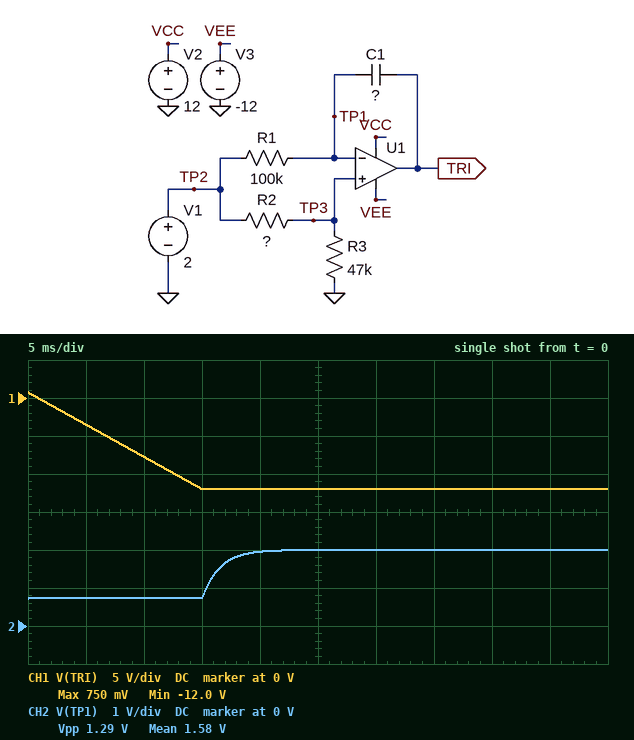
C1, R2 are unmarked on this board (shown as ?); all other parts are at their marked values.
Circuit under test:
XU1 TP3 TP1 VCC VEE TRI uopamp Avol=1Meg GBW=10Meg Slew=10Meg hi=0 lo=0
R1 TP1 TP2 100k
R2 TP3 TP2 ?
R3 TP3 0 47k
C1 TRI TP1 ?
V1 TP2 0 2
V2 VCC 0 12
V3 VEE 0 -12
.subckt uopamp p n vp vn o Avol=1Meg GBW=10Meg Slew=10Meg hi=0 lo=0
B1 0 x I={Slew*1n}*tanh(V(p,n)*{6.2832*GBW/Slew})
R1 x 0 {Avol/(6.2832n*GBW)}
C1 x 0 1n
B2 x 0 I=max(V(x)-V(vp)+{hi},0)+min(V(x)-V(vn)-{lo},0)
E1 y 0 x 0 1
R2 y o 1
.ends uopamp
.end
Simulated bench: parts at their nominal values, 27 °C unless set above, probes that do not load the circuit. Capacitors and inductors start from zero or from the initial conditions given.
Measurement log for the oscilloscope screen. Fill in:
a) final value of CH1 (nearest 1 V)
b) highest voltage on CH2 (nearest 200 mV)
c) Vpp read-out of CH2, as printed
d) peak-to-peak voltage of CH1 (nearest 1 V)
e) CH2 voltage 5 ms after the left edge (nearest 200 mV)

-12 V
2.0 V
1.29 V
13 V
800 mV
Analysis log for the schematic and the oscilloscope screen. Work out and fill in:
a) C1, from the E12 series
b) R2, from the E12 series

15 nF
82 kΩ
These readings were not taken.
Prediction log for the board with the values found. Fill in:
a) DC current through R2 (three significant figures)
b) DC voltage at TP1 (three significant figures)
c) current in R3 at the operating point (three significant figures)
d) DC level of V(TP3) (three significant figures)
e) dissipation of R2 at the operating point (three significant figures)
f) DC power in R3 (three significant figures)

15.5 µA
2.00 V
15.5 µA
729 mV
19.7 µW
11.3 µW
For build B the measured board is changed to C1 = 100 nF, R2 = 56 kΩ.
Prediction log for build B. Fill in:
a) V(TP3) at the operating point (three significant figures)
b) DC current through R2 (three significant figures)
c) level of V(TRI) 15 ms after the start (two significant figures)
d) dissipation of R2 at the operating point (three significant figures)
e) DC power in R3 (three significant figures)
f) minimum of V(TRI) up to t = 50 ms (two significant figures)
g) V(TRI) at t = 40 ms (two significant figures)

913 mV
19.4 µA
-720 mV
21.1 µW
17.7 µW
-4.5 V
-3.4 V
